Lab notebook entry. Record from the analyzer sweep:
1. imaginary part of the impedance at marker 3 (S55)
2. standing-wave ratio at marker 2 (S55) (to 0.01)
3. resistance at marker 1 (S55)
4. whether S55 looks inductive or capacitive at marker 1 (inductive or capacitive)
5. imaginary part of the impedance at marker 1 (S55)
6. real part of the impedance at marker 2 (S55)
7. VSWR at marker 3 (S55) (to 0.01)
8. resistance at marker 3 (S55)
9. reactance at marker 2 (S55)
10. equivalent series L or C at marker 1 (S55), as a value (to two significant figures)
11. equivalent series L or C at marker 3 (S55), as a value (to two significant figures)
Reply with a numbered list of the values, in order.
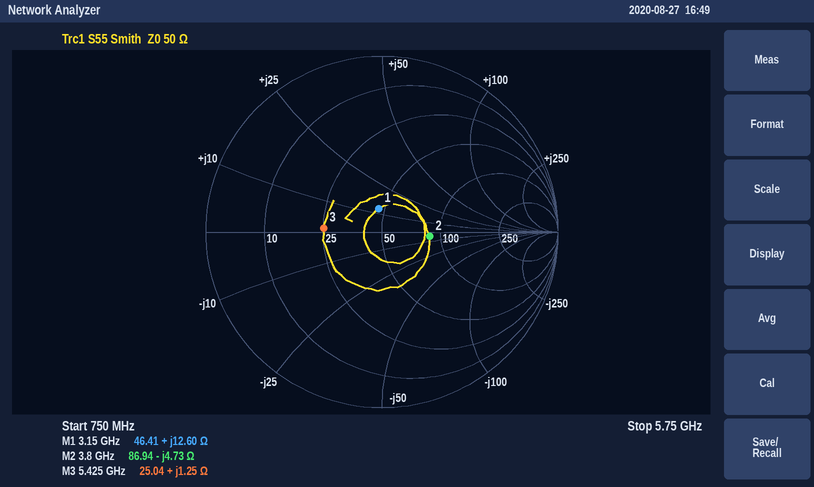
1. +1.25 Ω
2. 1.75
3. 46.41 Ω
4. inductive
5. +12.60 Ω
6. 86.94 Ω
7. 2.00
8. 25.04 Ω
9. -4.73 Ω
10. 640 pH
11. 37 pH
